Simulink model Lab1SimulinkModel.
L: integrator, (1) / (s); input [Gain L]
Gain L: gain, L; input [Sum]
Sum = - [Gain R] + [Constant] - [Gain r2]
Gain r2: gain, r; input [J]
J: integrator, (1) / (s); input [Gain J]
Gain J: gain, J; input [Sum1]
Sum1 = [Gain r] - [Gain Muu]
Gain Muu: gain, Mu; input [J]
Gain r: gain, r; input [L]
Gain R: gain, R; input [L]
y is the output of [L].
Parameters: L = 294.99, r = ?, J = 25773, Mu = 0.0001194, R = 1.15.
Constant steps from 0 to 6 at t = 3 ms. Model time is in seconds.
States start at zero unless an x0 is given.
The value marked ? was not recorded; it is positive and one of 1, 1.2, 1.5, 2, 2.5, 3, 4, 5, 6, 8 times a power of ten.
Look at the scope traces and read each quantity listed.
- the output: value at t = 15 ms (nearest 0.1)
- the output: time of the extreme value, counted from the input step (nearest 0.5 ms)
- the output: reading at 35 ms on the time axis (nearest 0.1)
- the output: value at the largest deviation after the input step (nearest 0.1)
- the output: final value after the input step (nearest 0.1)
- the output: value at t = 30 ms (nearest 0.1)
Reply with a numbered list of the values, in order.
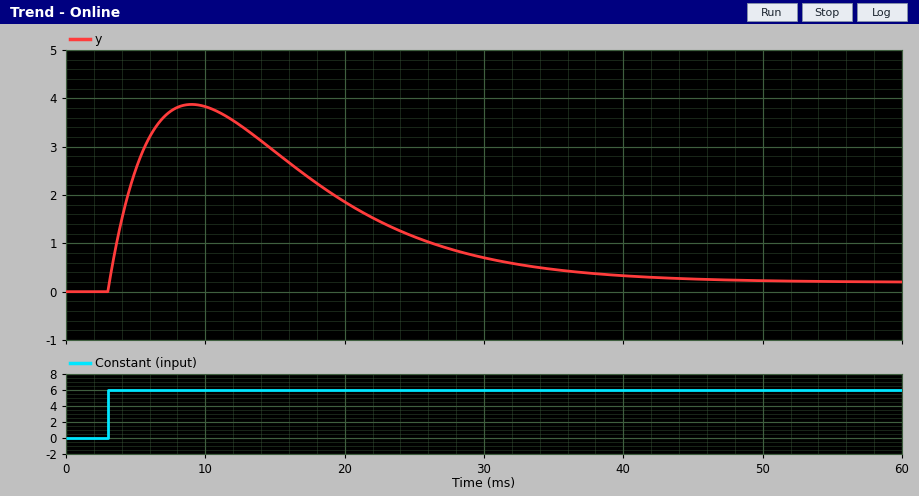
1. 2.9
2. 6.0 ms
3. 0.5
4. 3.9
5. 0.2
6. 0.7
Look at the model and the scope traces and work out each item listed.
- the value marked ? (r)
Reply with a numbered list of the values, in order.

1. 0.06
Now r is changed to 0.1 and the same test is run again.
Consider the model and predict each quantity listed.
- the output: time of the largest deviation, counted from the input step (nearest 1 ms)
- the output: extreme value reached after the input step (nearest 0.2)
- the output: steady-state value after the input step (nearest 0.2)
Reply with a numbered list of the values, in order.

1. 4 ms
2. 3.2
3. 0.0
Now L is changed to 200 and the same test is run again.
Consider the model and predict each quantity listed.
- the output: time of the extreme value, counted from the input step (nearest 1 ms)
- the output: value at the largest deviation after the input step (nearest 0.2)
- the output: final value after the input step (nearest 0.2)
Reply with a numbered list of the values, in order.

1. 8 ms
2. 3.6
3. 0.2
